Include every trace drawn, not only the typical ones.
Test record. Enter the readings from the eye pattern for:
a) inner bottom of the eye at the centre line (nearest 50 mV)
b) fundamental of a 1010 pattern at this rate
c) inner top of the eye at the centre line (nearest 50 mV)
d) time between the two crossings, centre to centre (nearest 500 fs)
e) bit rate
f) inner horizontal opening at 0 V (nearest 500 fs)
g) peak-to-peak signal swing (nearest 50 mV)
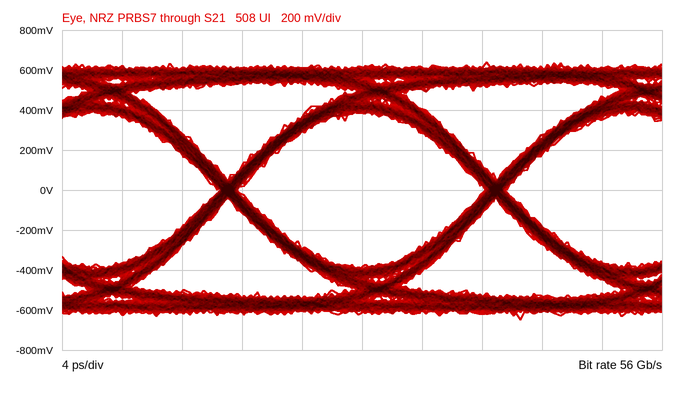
-400 mV
28 GHz
400 mV
18.0 ps
56 Gb/s
16.5 ps
1.30 V
